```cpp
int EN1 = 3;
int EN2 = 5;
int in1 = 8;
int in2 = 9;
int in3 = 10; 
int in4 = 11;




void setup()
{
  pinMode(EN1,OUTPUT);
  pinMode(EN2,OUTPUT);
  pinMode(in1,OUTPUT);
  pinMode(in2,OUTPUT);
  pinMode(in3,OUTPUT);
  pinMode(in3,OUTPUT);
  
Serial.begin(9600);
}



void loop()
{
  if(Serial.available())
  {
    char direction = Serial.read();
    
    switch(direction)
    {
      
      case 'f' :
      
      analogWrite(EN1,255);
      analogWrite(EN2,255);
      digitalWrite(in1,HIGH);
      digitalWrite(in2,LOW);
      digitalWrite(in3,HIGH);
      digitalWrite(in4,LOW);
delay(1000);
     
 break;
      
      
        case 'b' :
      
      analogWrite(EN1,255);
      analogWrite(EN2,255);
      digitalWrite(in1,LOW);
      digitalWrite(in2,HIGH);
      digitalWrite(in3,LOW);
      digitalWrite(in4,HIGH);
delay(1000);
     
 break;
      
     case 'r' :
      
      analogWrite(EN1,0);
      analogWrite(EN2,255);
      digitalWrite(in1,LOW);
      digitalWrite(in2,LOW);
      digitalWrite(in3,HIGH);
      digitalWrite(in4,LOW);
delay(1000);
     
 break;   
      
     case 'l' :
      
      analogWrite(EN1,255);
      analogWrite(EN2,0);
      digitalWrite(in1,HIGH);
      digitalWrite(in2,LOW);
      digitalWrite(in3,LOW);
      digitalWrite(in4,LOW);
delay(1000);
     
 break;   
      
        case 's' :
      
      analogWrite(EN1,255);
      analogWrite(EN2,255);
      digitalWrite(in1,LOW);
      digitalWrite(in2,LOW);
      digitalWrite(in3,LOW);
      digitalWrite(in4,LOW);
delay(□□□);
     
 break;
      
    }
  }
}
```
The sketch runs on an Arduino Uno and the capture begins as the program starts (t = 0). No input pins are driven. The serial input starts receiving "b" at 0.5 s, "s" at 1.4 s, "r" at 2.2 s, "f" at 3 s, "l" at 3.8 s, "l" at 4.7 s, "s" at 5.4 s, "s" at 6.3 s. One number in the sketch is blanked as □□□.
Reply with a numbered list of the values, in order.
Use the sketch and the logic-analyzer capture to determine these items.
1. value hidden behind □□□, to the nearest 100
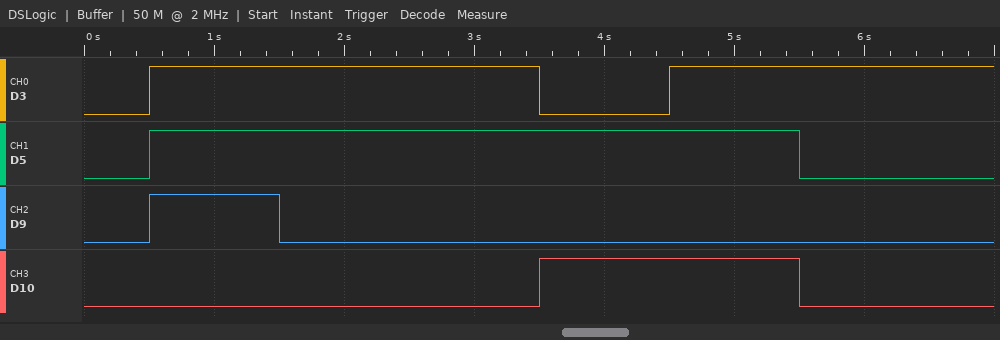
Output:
1. 2000
